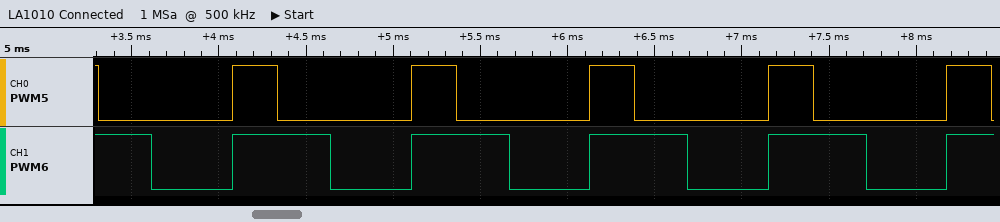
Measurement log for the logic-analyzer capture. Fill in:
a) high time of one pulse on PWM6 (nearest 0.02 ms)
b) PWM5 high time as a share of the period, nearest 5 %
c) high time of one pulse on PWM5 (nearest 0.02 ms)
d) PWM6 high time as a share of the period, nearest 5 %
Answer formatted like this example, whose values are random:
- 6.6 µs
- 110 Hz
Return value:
- 0.56 ms
- 25 %
- 0.26 ms
- 55 %
